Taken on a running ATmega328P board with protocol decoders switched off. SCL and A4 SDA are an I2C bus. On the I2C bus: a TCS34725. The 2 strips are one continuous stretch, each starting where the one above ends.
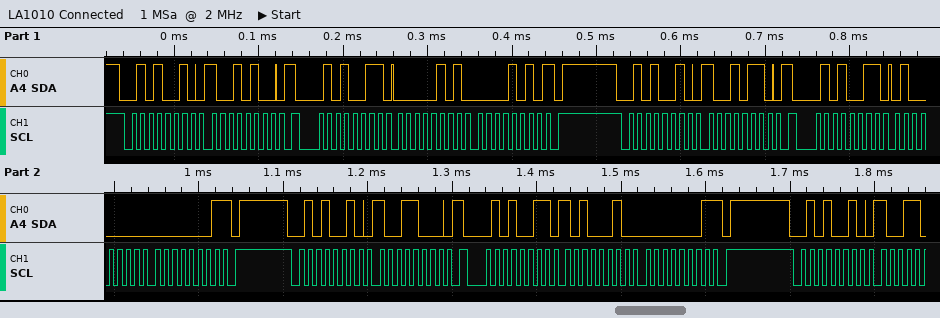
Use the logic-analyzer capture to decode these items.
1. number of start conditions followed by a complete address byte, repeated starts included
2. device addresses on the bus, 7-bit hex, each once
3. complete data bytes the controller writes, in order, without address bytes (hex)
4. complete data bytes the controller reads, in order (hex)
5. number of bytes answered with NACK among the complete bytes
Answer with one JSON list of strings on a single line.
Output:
["7", "0x29", "94 96 98", "05 0A 40 01 A2 01", "3"]
